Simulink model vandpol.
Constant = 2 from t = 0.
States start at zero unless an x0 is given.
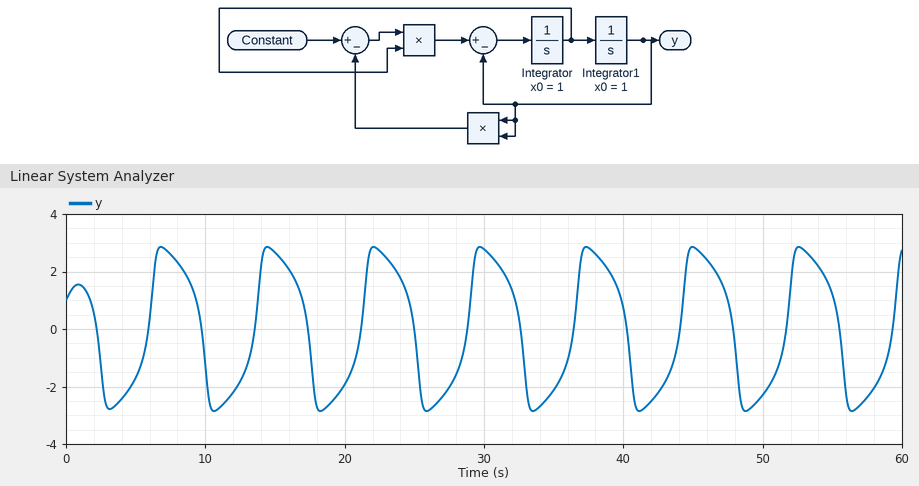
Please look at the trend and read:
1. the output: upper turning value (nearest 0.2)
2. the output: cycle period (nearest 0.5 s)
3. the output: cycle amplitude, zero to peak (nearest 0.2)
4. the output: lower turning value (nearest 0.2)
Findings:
2.8
7.5 s
2.8
-2.8
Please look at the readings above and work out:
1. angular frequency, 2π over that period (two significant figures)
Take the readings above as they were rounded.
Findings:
0.84 rad/s
